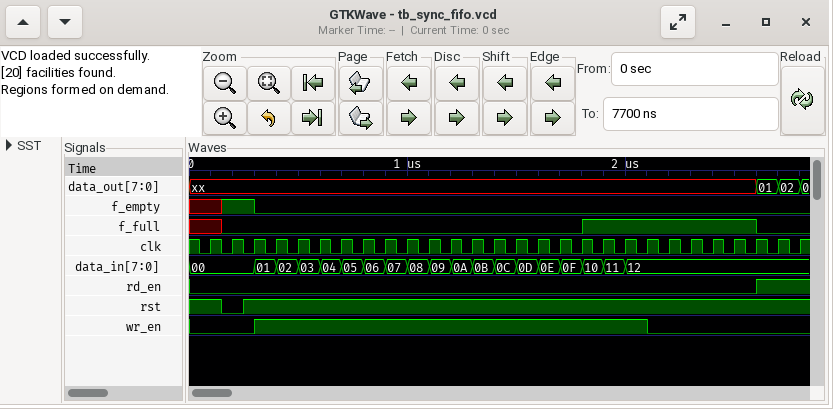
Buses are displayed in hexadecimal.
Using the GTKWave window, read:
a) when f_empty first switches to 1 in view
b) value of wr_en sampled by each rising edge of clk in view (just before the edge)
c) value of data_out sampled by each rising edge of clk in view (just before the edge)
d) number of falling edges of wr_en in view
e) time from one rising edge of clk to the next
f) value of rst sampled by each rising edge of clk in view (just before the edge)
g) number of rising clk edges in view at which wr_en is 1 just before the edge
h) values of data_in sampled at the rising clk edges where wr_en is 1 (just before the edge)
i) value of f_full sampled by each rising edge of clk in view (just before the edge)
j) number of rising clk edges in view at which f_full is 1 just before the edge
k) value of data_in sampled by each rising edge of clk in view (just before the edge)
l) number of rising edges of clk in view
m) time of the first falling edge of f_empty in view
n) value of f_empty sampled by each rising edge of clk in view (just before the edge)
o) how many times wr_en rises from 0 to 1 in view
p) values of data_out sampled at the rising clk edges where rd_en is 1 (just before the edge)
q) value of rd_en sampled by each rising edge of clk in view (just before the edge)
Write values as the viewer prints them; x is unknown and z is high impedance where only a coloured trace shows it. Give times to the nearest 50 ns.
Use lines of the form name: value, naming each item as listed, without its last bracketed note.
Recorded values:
when f_empty first switches to 1 in view: 150 ns
value of wr_en sampled by each rising edge of clk in view: 0 0 0 1 1 1 1 1 1 1 1 1 1 1 1 1 1 1 1 1 1 0 0 0 0 0 0 0
value of data_out sampled by each rising edge of clk in view: xx, xx, xx, xx, xx, xx, xx, xx, xx, xx, xx, xx, xx, xx, xx, xx, xx, xx, xx, xx, xx, xx, xx, xx, xx, xx, 01, 02
number of falling edges of wr_en in view: 1
time from one rising edge of clk to the next: 100 ns
value of rst sampled by each rising edge of clk in view: 1 0 1 1 1 1 1 1 1 1 1 1 1 1 1 1 1 1 1 1 1 1 1 1 1 1 1 1
number of rising clk edges in view at which wr_en is 1 just before the edge: 18
values of data_in sampled at the rising clk edges where wr_en is 1: 01, 02, 03, 04, 05, 06, 07, 08, 09, 0A, 0B, 0C, 0D, 0E, 0F, 10, 11, 12
value of f_full sampled by each rising edge of clk in view: x 0 0 0 0 0 0 0 0 0 0 0 0 0 0 0 0 0 1 1 1 1 1 1 1 1 0 0
number of rising clk edges in view at which f_full is 1 just before the edge: 8
value of data_in sampled by each rising edge of clk in view: 00, 00, 00, 01, 02, 03, 04, 05, 06, 07, 08, 09, 0A, 0B, 0C, 0D, 0E, 0F, 10, 11, 12, 12, 12, 12, 12, 12, 12, 12
number of rising edges of clk in view: 28
time of the first falling edge of f_empty in view: 300 ns
value of f_empty sampled by each rising edge of clk in view: x 1 1 0 0 0 0 0 0 0 0 0 0 0 0 0 0 0 0 0 0 0 0 0 0 0 0 0
how many times wr_en rises from 0 to 1 in view: 1
values of data_out sampled at the rising clk edges where rd_en is 1: 01, 02
value of rd_en sampled by each rising edge of clk in view: 0 0 0 0 0 0 0 0 0 0 0 0 0 0 0 0 0 0 0 0 0 0 0 0 0 0 1 1
